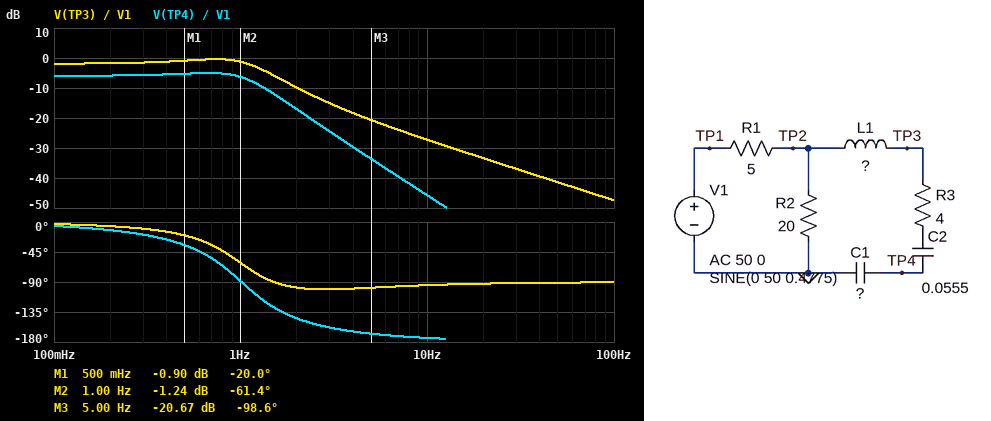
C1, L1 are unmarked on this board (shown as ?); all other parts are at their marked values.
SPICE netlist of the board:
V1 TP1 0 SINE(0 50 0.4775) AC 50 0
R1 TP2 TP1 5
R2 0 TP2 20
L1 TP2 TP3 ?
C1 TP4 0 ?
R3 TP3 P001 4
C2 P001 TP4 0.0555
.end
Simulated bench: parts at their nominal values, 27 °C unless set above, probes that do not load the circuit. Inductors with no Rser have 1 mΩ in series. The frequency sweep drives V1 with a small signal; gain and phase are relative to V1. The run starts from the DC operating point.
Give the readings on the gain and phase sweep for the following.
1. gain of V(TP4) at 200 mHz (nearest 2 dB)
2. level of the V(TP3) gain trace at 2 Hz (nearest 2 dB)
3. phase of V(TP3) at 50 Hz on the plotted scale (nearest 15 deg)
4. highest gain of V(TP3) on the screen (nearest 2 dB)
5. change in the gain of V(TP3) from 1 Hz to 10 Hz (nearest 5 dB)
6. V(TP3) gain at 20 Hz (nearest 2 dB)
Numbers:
-6 dB
-10 dB
-90 deg
0 dB
-25 dB
-34 dB
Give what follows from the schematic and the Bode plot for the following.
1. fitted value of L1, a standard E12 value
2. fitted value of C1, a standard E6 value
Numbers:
1.2 H
33 mF
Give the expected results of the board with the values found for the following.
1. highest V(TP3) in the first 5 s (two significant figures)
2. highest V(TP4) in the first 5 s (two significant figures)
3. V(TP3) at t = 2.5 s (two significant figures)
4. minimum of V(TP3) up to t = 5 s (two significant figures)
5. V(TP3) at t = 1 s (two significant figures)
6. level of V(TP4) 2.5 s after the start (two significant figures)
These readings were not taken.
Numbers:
45 V
27 V
35 V
-45 V
21 V
16 V
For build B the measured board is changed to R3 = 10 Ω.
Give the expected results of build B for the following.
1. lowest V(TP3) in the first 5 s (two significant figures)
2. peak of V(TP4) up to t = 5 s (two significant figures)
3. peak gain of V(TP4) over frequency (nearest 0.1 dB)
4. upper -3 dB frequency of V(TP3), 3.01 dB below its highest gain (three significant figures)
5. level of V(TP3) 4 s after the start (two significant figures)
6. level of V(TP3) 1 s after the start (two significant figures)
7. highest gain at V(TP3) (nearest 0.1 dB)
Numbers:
-40 V
22 V
-6.0 dB
1.56 Hz
-30 V
17 V
-1.8 dB
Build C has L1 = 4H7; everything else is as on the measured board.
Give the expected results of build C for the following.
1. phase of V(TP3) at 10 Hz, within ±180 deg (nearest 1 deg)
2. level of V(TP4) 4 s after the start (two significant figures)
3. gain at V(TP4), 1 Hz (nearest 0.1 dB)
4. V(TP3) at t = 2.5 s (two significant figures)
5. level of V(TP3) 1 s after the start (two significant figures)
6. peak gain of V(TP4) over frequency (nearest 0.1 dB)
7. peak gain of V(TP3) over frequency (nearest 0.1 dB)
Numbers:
-99 deg
-45 V
-15.6 dB
9.9 V
45 V
-0.2 dB
4.1 dB
